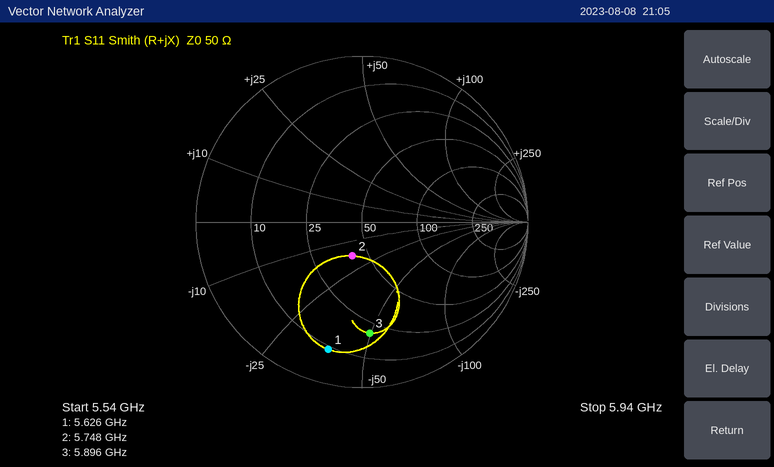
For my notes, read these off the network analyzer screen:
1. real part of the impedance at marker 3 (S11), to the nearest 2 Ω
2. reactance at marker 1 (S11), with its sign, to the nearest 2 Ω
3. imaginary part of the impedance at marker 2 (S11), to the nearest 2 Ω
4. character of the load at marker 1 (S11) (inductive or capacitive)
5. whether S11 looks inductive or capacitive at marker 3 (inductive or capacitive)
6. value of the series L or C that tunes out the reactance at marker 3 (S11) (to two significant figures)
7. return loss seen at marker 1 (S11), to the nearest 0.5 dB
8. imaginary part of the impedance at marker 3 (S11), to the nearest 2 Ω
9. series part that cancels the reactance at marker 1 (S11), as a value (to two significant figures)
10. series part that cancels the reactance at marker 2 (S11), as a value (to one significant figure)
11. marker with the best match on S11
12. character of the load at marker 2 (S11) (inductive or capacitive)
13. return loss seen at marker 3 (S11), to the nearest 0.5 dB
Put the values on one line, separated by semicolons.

20 Ω; -38 Ω; -18 Ω; capacitive; capacitive; 1.3 nH; 2.0 dB; -50 Ω; 1.1 nH; 500 pH; marker 2; capacitive; 3.5 dB
